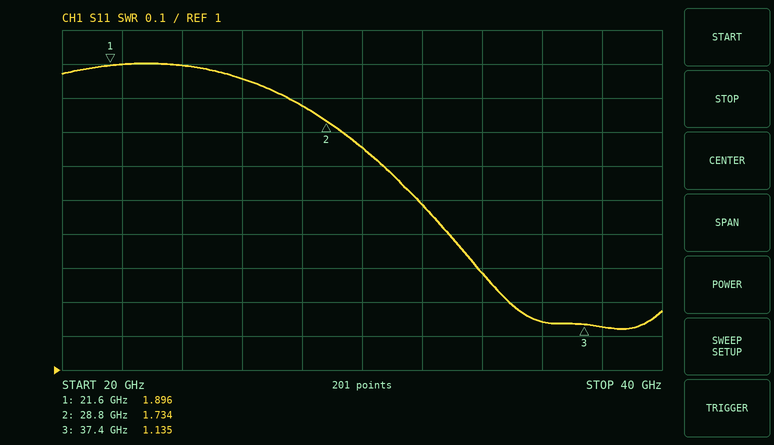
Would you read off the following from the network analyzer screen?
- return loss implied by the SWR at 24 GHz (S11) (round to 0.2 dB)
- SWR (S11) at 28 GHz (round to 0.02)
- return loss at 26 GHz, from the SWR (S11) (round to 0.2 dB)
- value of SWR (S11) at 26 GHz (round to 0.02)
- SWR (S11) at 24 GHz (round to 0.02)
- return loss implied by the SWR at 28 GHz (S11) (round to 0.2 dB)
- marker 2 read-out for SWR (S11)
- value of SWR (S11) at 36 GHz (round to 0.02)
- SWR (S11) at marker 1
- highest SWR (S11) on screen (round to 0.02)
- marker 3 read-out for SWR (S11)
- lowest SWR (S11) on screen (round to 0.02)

10.2 dB
1.78
10.4 dB
1.86
1.90
11.0 dB
1.734
1.14
1.896
1.90
1.135
1.12
